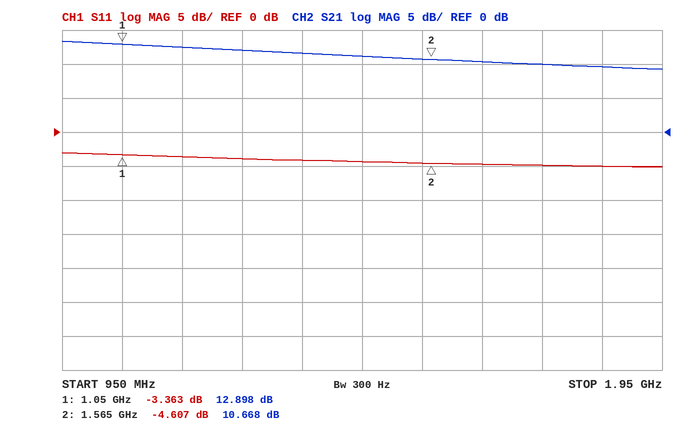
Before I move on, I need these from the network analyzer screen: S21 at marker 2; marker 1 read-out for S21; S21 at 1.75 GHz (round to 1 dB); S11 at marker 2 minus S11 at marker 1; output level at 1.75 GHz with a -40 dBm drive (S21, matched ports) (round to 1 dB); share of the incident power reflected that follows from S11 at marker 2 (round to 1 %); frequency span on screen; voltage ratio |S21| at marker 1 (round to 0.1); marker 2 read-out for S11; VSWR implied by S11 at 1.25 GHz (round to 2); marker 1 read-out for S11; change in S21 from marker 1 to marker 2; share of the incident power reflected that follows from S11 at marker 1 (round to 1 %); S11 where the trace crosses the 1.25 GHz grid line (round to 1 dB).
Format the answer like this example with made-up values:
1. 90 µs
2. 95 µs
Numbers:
1. 10.668 dB
2. 12.898 dB
3. 10 dB
4. -1.244 dB
5. -30 dBm
6. 35 %
7. 1 GHz
8. 4.4
9. -4.607 dB
10. 4
11. -3.363 dB
12. -2.230 dB
13. 46 %
14. -4 dB
